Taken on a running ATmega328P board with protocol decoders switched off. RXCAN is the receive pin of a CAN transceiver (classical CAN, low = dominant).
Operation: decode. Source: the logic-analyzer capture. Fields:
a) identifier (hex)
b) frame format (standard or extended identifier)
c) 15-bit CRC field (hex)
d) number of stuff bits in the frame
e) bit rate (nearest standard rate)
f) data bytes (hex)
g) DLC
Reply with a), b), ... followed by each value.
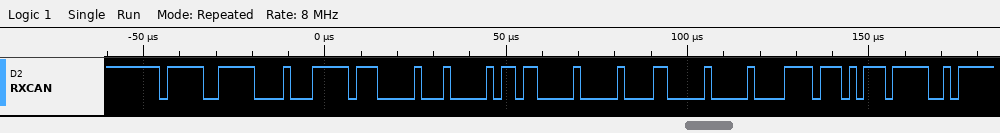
a) 0x7DF
b) standard
c) 0x6BBE
d) 10
e) 500 kbit/s
f) FF 00 81 B0 00 30 00 3D
g) 8
